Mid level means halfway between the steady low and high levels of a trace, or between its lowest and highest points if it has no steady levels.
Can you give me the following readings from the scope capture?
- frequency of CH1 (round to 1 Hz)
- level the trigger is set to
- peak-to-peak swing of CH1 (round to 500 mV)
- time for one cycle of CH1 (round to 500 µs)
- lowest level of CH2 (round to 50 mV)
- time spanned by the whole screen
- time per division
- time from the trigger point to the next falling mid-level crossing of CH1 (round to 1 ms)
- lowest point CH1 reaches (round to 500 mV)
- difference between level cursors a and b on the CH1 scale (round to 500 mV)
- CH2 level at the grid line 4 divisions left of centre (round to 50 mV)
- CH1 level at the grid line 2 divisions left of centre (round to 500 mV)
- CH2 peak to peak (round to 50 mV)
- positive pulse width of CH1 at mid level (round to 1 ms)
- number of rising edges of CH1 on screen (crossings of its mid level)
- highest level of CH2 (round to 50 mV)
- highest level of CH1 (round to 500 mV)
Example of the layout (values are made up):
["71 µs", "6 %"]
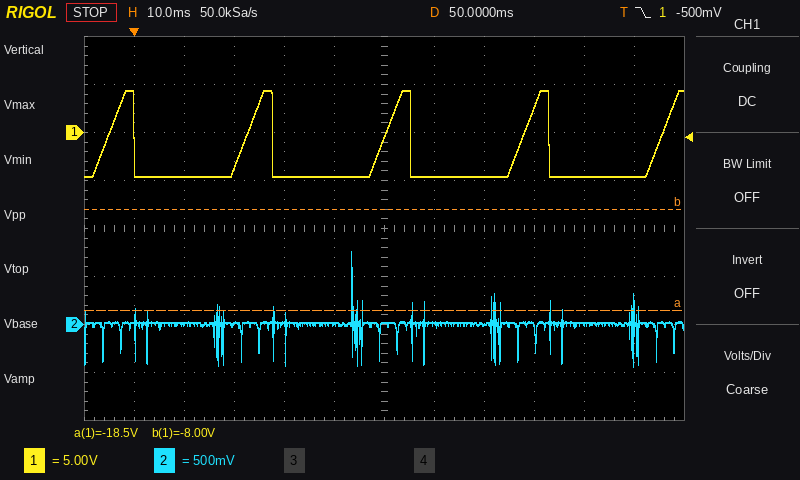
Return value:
["36 Hz", "-500 mV", "9.0 V", "27.5 ms", "-450 mV", "120 ms", "10 ms", "28 ms", "-4.5 V", "10.5 V", "0 mV", "-4.5 V", "1.20 V", "5 ms", "5", "750 mV", "4.5 V"]
